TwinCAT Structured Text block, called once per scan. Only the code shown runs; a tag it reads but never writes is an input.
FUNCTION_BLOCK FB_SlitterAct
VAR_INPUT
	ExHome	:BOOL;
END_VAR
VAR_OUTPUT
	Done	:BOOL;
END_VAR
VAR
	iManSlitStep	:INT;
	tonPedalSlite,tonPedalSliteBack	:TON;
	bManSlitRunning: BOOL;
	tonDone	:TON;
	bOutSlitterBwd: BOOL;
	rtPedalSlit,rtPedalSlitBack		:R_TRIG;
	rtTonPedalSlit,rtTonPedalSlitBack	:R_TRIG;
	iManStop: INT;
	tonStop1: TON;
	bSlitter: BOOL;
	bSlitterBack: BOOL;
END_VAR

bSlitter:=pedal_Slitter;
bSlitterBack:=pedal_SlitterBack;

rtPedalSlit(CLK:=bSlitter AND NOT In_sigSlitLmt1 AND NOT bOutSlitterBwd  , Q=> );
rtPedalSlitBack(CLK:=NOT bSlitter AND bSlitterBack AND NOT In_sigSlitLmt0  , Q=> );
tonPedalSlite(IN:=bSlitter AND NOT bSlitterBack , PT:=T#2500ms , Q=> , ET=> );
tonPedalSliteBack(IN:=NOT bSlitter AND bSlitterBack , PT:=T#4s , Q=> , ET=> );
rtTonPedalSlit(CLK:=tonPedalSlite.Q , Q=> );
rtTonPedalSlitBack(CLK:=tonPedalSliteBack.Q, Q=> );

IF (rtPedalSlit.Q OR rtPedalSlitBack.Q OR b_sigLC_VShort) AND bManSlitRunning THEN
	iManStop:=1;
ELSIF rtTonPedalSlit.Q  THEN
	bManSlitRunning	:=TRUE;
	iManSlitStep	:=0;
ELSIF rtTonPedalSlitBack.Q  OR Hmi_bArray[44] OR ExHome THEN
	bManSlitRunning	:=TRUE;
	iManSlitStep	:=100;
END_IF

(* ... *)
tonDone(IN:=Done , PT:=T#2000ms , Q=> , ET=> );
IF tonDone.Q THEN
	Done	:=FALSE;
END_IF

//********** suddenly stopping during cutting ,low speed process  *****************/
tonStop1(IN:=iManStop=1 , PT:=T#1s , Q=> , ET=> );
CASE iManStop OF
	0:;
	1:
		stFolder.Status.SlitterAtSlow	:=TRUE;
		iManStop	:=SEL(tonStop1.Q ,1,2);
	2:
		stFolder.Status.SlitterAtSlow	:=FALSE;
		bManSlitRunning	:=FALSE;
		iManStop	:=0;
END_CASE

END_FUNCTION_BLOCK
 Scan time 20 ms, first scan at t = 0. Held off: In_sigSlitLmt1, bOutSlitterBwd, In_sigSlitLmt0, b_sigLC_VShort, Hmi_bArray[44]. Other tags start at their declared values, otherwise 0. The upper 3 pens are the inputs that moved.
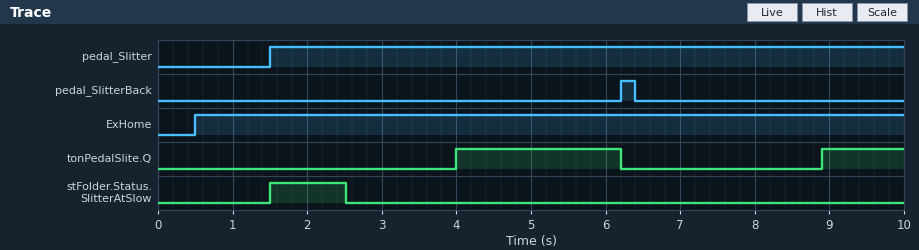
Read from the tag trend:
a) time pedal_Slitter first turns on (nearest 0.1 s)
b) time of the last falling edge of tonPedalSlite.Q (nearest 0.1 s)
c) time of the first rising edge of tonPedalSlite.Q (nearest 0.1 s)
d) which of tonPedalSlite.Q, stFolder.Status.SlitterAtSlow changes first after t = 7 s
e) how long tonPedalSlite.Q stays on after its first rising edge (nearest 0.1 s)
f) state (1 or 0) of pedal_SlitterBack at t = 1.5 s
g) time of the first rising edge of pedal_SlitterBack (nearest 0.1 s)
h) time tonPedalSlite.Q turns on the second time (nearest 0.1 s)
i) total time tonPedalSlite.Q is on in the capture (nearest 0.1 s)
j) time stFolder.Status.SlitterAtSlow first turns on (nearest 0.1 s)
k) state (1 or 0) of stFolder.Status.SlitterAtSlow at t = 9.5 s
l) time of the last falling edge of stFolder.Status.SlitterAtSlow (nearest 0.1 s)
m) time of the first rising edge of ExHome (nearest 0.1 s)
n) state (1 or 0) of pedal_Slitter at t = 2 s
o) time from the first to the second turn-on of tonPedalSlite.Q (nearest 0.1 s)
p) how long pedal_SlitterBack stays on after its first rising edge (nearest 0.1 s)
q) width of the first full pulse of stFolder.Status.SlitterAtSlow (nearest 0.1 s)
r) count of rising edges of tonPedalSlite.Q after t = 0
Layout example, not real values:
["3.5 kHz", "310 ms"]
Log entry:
["1.5 s", "6.2 s", "4.0 s", "tonPedalSlite.Q", "2.2 s", "0", "6.2 s", "8.9 s", "3.3 s", "1.5 s", "0", "2.5 s", "0.5 s", "1", "4.9 s", "0.2 s", "1.0 s", "2"]
